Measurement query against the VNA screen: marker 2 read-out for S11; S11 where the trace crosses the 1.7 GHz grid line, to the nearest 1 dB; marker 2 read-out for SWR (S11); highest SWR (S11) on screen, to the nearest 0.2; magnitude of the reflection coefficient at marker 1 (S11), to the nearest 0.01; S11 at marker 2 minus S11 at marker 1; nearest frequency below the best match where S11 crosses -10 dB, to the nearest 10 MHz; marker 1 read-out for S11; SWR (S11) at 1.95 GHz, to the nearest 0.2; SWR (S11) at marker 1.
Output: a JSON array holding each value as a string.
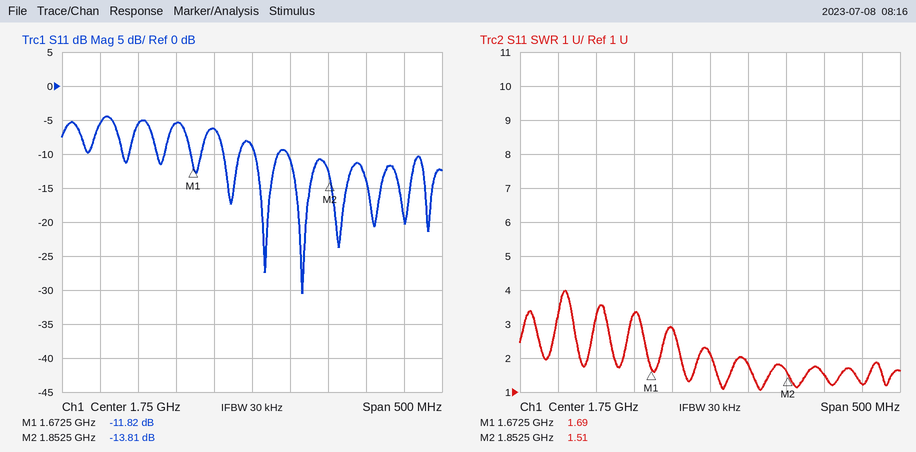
["-13.81 dB", "-6 dB", "1.51", "4.0", "0.26", "-1.99 dB", "1.80 GHz", "-11.82 dB", "1.2", "1.69"]
